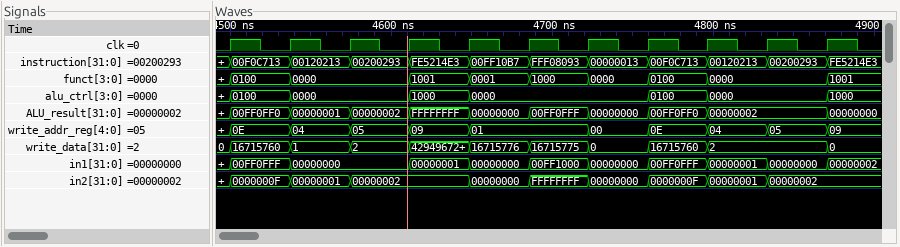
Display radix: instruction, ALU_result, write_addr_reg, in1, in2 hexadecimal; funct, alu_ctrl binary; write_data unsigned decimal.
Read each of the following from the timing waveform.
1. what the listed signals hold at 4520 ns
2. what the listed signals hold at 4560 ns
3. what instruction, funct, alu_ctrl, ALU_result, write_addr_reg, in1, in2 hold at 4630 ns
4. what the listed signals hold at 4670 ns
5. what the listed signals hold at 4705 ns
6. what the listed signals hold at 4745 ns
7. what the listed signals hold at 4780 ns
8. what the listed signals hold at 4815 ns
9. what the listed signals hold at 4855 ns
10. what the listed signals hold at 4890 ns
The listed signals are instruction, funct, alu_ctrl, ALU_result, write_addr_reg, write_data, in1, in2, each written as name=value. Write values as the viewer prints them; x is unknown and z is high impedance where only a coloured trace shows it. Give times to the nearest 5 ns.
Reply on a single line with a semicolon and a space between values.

instruction=00F0C713, funct=0100, alu_ctrl=0100, ALU_result=00FF0FF0, write_addr_reg=0E, write_data=16715760, in1=00FF0FFF, in2=0000000F; instruction=00120213, funct=0000, alu_ctrl=0000, ALU_result=00000001, write_addr_reg=04, write_data=1, in1=00000000, in2=00000001; instruction=FE5214E3, funct=1001, alu_ctrl=1000, ALU_result=FFFFFFFF, write_addr_reg=09, in1=00000001, in2=00000002; instruction=00FF10B7, funct=0001, alu_ctrl=0000, ALU_result=00000000, write_addr_reg=01, write_data=16715776, in1=00000000, in2=00000000; instruction=FFF08093, funct=1000, alu_ctrl=0000, ALU_result=00FF0FFF, write_addr_reg=01, write_data=16715775, in1=00FF1000, in2=FFFFFFFF; instruction=00000013, funct=0000, alu_ctrl=0000, ALU_result=00000000, write_addr_reg=00, write_data=0, in1=00000000, in2=00000000; instruction=00F0C713, funct=0100, alu_ctrl=0100, ALU_result=00FF0FF0, write_addr_reg=0E, write_data=16715760, in1=00FF0FFF, in2=0000000F; instruction=00120213, funct=0000, alu_ctrl=0000, ALU_result=00000002, write_addr_reg=04, write_data=2, in1=00000001, in2=00000001; instruction=00200293, funct=0000, alu_ctrl=0000, ALU_result=00000002, write_addr_reg=05, write_data=2, in1=00000000, in2=00000002; instruction=FE5214E3, funct=1001, alu_ctrl=1000, ALU_result=00000000, write_addr_reg=09, write_data=0, in1=00000002, in2=00000002
